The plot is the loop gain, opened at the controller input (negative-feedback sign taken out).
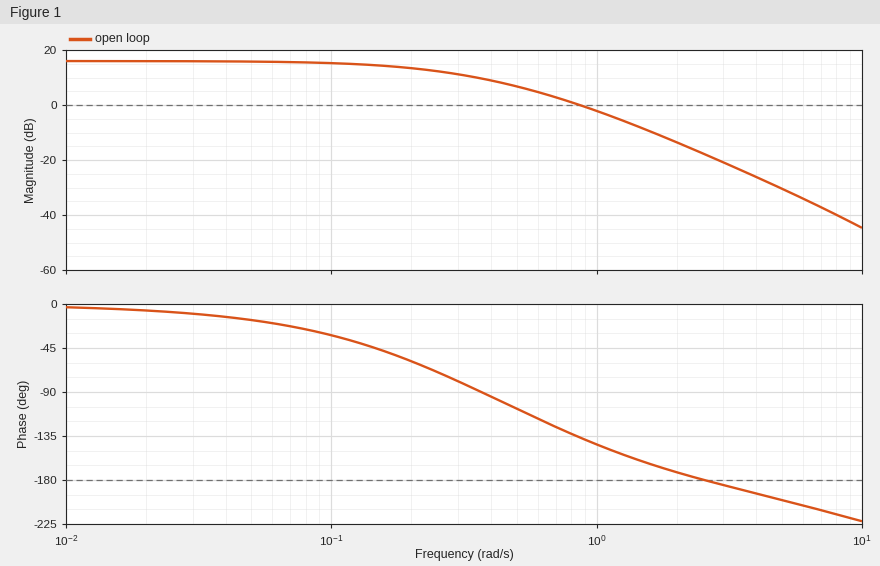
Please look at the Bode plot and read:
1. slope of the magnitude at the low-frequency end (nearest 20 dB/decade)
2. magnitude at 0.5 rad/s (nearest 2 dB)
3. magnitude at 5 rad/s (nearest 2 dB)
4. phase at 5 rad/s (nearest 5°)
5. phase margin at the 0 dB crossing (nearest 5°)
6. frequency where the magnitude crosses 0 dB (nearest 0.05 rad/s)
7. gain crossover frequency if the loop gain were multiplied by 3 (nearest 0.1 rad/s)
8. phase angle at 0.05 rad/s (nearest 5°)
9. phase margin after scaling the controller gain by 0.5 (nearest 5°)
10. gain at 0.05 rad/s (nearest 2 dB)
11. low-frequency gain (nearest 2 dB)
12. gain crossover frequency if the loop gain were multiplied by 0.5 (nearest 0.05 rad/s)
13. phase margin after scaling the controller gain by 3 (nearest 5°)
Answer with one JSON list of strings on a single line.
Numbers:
["0 dB/decade", "6 dB", "-30 dB", "-200°", "45°", "0.85 rad/s", "1.6 rad/s", "-15°", "70°", "16 dB", "16 dB", "0.55 rad/s", "15°"]
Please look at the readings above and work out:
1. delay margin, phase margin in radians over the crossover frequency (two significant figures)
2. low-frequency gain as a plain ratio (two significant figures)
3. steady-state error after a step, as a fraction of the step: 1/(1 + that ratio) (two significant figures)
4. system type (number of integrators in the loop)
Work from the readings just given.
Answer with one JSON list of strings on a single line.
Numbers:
["0.92 s", "6.3", "0.14", "0"]
